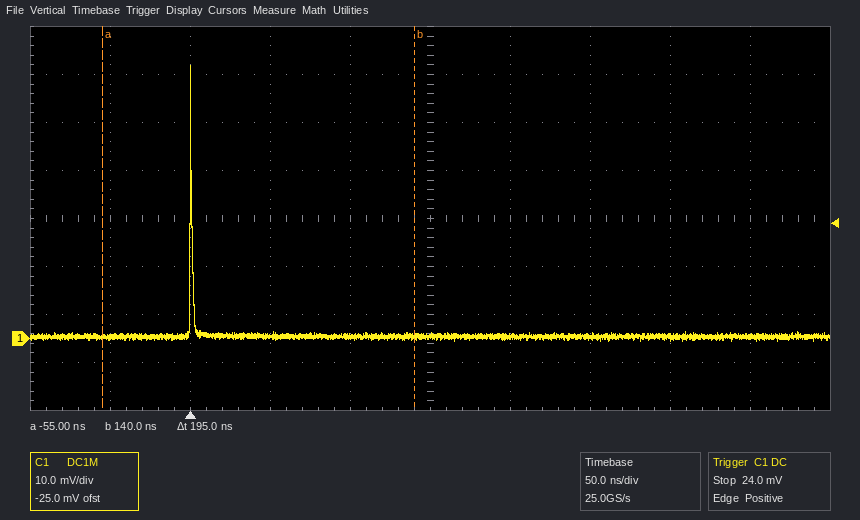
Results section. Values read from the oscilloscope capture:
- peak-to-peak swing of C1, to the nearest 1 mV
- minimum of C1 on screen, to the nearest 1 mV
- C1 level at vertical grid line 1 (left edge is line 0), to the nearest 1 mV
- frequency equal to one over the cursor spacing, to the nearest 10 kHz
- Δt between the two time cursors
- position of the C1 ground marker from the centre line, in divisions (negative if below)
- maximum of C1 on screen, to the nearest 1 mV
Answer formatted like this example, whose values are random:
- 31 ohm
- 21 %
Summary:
- 57 mV
- 0 mV
- 0 mV
- 5.13 MHz
- 195 ns
- -2.5 div
- 57 mV
